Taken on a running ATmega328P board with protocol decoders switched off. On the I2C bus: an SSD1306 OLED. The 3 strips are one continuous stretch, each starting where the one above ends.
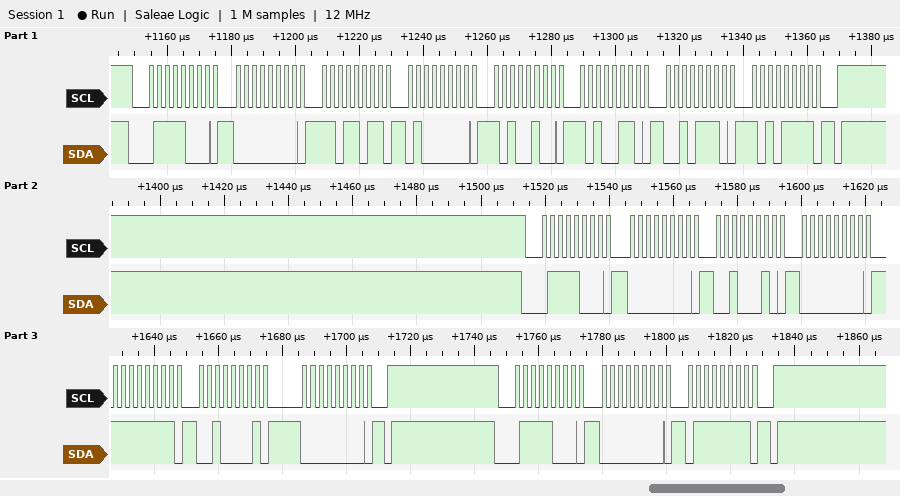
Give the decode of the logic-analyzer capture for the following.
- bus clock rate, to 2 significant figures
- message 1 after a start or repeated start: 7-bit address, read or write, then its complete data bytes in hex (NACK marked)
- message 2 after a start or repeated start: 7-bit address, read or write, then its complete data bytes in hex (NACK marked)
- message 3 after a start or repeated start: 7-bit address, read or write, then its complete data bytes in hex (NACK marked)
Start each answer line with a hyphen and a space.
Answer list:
- 400 kHz
- 0x3C write: 00 DB 40 A4 A6 2E AF
- 0x3C write: 00 22 00 FF 21 00
- 0x3C write: 00 7F
